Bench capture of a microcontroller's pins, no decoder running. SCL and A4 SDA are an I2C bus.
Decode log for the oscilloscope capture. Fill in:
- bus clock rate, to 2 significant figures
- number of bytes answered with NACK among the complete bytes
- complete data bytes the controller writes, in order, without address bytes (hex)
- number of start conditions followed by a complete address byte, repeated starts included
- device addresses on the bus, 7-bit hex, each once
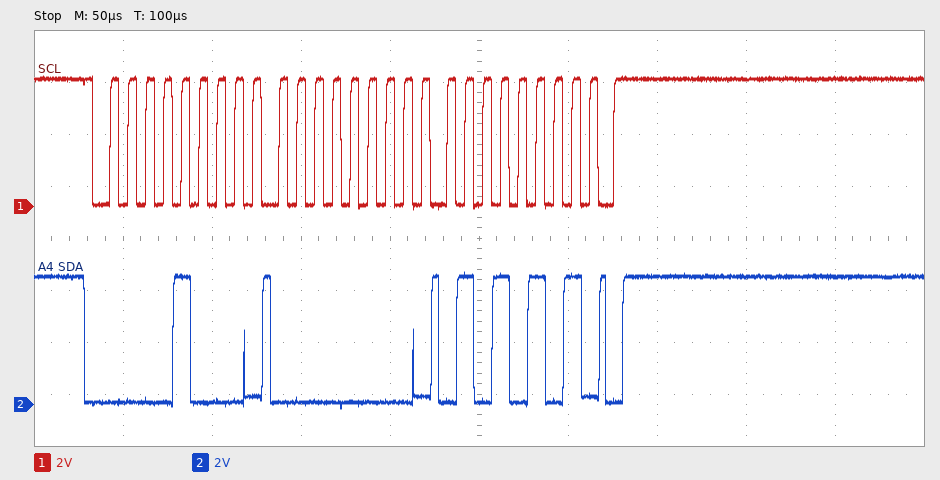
100 kHz
0
00 55
1
0x04
